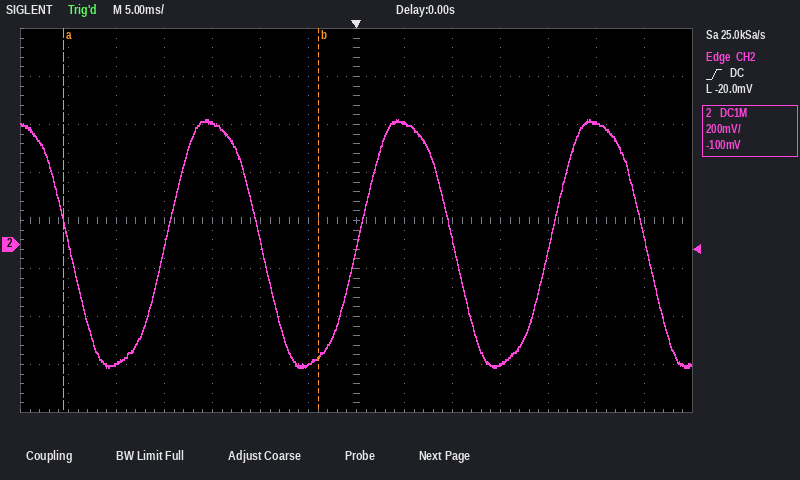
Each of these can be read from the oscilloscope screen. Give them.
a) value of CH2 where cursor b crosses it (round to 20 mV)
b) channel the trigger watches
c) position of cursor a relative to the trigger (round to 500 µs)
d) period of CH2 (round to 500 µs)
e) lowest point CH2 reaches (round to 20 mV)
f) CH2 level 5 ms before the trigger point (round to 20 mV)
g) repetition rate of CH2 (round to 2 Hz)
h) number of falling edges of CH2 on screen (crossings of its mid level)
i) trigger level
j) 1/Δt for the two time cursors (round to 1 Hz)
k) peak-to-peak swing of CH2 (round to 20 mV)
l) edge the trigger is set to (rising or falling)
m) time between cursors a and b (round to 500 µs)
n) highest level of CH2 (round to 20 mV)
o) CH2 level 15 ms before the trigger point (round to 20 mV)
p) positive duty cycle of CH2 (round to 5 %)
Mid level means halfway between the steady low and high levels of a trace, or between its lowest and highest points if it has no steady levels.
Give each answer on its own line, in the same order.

-460 mV
CH2
-30.5 ms
20.0 ms
-520 mV
-500 mV
50 Hz
4
-20.0 mV
38 Hz
1.04 V
rising
26.5 ms
520 mV
500 mV
50 %
